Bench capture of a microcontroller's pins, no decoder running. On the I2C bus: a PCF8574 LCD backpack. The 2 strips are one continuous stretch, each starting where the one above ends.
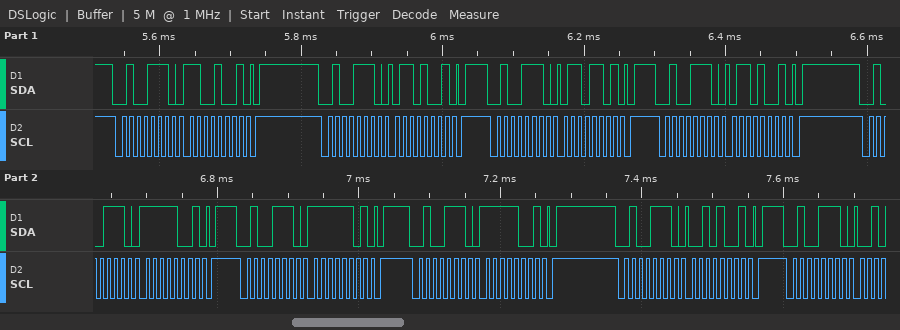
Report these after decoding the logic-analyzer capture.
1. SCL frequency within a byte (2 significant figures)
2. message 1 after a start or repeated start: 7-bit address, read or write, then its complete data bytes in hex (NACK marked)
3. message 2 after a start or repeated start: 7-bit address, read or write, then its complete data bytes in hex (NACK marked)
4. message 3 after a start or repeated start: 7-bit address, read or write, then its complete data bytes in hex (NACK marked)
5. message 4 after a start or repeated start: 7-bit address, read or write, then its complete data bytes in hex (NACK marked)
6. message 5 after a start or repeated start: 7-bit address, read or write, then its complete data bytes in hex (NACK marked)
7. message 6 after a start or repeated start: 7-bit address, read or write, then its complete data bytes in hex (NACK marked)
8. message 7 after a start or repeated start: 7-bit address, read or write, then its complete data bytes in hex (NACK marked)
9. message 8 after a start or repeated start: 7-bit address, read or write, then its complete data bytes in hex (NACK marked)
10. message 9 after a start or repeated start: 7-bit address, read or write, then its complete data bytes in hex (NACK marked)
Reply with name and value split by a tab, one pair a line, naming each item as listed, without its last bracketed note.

SCL frequency within a byte	100 kHz
message 1 after a start or repeated start: 7-bit address, read or write, then its complete data bytes in hex	0x27 write: C9
message 2 after a start or repeated start: 7-bit address, read or write, then its complete data bytes in hex	0x27 write: 69
message 3 after a start or repeated start: 7-bit address, read or write, then its complete data bytes in hex	0x27 write: 6D
message 4 after a start or repeated start: 7-bit address, read or write, then its complete data bytes in hex	0x27 write: 69
message 5 after a start or repeated start: 7-bit address, read or write, then its complete data bytes in hex	0x27 write: F9
message 6 after a start or repeated start: 7-bit address, read or write, then its complete data bytes in hex	0x27 write: FD
message 7 after a start or repeated start: 7-bit address, read or write, then its complete data bytes in hex	0x27 write: F9
message 8 after a start or repeated start: 7-bit address, read or write, then its complete data bytes in hex	0x27 write: 29
message 9 after a start or repeated start: 7-bit address, read or write, then its complete data bytes in hex	0x27 write
